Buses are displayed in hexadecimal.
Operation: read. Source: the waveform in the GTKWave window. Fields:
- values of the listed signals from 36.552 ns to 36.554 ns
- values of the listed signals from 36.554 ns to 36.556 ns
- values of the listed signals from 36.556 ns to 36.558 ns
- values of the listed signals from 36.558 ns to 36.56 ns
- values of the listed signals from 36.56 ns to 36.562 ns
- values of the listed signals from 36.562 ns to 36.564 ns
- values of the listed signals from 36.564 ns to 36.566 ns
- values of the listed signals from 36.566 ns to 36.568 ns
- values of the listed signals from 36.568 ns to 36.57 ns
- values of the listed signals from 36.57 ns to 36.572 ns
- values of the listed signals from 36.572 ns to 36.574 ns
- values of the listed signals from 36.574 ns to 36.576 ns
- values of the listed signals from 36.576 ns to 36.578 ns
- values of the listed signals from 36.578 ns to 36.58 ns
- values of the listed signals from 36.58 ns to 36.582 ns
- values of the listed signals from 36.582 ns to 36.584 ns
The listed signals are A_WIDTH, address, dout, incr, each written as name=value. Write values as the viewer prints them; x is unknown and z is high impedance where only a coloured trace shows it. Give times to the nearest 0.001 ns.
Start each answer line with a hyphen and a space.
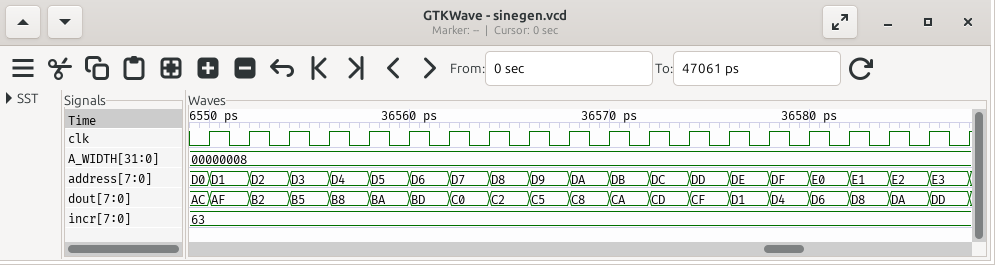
- A_WIDTH=00000008, address=D2, dout=B2, incr=63
- A_WIDTH=00000008, address=D3, dout=B5, incr=63
- A_WIDTH=00000008, address=D4, dout=B8, incr=63
- A_WIDTH=00000008, address=D5, dout=BA, incr=63
- A_WIDTH=00000008, address=D6, dout=BD, incr=63
- A_WIDTH=00000008, address=D7, dout=C0, incr=63
- A_WIDTH=00000008, address=D8, dout=C2, incr=63
- A_WIDTH=00000008, address=D9, dout=C5, incr=63
- A_WIDTH=00000008, address=DA, dout=C8, incr=63
- A_WIDTH=00000008, address=DB, dout=CA, incr=63
- A_WIDTH=00000008, address=DC, dout=CD, incr=63
- A_WIDTH=00000008, address=DD, dout=CF, incr=63
- A_WIDTH=00000008, address=DE, dout=D1, incr=63
- A_WIDTH=00000008, address=DF, dout=D4, incr=63
- A_WIDTH=00000008, address=E0, dout=D6, incr=63
- A_WIDTH=00000008, address=E1, dout=D8, incr=63
